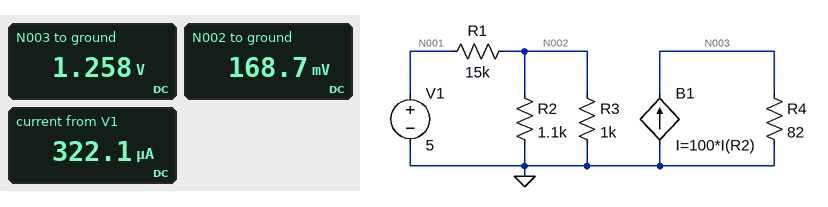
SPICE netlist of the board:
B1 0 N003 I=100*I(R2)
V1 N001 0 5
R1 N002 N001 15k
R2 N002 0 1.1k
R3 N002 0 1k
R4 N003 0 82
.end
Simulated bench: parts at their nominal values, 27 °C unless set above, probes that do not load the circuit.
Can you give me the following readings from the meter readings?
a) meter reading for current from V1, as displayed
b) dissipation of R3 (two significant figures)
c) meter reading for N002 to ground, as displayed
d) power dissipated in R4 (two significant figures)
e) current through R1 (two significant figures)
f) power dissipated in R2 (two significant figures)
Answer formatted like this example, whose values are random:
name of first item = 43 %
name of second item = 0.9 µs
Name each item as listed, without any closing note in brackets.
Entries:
meter reading for current from V1, as displayed = 322.1 µA
dissipation of R3 = 28 µW
meter reading for N002 to ground, as displayed = 168.7 mV
power dissipated in R4 = 19 mW
current through R1 = 320 µA
power dissipated in R2 = 26 µW
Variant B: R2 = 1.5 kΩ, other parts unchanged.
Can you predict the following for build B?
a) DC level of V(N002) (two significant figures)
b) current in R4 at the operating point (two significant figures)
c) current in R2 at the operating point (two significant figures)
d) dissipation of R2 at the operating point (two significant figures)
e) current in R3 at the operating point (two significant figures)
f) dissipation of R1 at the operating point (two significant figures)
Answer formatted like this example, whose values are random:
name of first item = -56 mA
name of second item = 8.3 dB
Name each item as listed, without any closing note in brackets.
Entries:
DC level of V(N002) = 190 mV
current in R4 at the operating point = 13 mA
current in R2 at the operating point = 130 µA
dissipation of R2 at the operating point = 25 µW
current in R3 at the operating point = 190 µA
dissipation of R1 at the operating point = 1.5 mW
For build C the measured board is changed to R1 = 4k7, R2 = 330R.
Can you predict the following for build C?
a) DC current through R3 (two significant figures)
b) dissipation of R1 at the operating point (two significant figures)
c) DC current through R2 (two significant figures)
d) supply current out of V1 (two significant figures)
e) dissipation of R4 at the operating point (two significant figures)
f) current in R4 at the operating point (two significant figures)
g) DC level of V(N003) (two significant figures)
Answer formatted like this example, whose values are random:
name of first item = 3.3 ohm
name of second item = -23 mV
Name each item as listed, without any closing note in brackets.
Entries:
DC current through R3 = 250 µA
dissipation of R1 at the operating point = 4.8 mW
DC current through R2 = 760 µA
supply current out of V1 = 1.0 mA
dissipation of R4 at the operating point = 470 mW
current in R4 at the operating point = 76 mA
DC level of V(N003) = 6.2 V
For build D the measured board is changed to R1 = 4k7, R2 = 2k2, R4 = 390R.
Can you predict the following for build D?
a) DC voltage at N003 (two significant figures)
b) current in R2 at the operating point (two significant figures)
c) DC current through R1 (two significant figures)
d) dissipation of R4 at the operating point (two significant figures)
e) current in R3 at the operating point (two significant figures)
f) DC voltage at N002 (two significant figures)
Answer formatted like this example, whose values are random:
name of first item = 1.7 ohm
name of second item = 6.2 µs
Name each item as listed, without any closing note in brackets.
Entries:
DC voltage at N003 = 11 V
current in R2 at the operating point = 290 µA
DC current through R1 = 930 µA
dissipation of R4 at the operating point = 330 mW
current in R3 at the operating point = 640 µA
DC voltage at N002 = 640 mV
